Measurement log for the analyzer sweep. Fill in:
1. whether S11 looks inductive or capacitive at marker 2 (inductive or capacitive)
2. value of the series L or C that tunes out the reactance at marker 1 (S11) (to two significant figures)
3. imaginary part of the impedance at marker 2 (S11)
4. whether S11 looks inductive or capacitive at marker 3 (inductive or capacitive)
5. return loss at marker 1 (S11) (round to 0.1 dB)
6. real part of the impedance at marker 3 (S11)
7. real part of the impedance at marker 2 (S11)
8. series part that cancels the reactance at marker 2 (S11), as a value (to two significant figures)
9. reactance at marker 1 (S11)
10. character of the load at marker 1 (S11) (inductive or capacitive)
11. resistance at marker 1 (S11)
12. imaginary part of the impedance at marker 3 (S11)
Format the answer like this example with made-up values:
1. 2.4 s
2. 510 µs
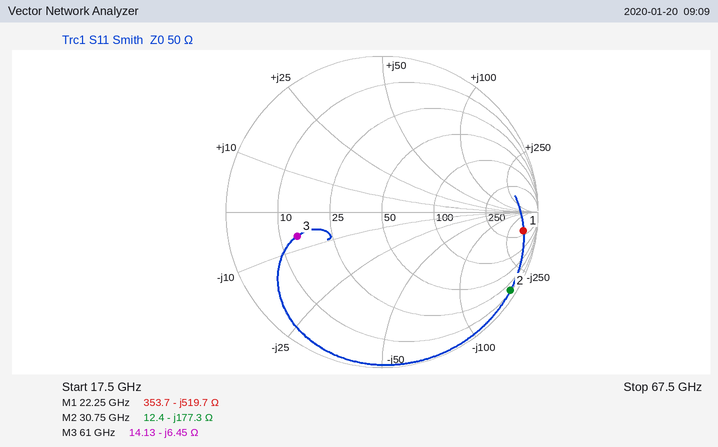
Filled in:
1. capacitive
2. 3.7 nH
3. -177.3 Ω
4. capacitive
5. 0.8 dB
6. 14.13 Ω
7. 12.4 Ω
8. 920 pH
9. -519.7 Ω
10. capacitive
11. 353.7 Ω
12. -6.45 Ω
